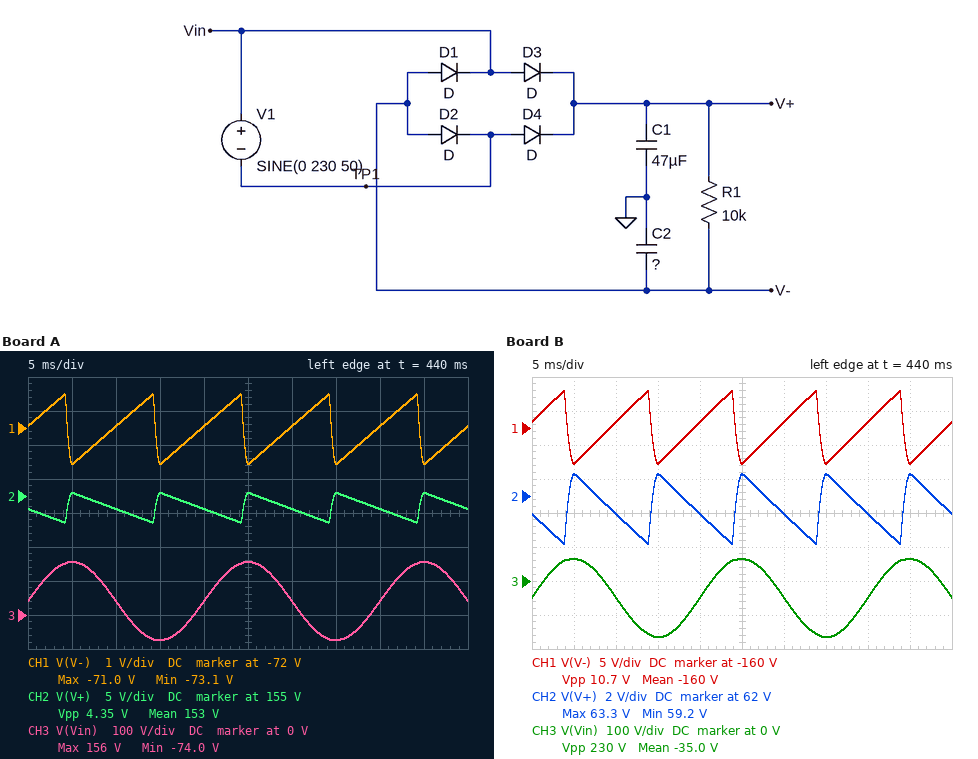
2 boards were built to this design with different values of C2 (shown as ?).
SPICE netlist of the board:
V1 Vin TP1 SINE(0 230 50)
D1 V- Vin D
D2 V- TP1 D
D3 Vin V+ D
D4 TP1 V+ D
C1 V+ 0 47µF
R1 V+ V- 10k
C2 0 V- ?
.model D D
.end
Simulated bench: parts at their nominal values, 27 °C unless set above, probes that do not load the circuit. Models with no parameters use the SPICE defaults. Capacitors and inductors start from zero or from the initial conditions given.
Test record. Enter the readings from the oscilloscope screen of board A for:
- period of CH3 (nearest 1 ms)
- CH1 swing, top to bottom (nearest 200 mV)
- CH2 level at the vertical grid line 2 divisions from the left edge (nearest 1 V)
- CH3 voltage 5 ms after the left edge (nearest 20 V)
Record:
20 ms
2.0 V
153 V
160 V
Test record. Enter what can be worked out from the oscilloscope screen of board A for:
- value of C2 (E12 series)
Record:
100 µF
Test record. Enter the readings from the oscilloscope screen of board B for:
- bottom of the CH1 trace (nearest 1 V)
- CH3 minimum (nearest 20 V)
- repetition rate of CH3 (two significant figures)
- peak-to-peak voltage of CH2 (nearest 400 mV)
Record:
-165 V
-160 V
50 Hz
4.0 V
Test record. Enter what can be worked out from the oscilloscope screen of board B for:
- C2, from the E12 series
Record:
18 µF
